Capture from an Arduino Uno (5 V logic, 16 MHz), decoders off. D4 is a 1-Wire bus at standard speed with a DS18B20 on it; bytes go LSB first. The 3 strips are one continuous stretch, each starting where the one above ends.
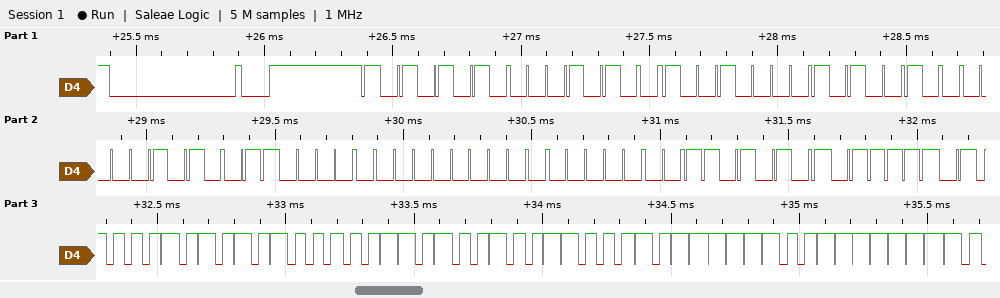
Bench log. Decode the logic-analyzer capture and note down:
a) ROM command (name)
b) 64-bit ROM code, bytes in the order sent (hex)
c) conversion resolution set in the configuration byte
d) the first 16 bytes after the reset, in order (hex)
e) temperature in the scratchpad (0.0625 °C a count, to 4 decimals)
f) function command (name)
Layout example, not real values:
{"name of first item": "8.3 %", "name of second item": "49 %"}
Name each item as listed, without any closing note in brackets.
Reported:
{"ROM command": "Match ROM", "64-bit ROM code, bytes in the order sent": "28 09 25 50 06 00 00 AB", "conversion resolution set in the configuration byte": "10 bits", "the first 16 bytes after the reset, in order": "55 28 09 25 50 06 00 00 AB BE 50 05 4B 46 3F FF", "temperature in the scratchpad": "85.0000 °C", "function command": "Read Scratchpad"}
